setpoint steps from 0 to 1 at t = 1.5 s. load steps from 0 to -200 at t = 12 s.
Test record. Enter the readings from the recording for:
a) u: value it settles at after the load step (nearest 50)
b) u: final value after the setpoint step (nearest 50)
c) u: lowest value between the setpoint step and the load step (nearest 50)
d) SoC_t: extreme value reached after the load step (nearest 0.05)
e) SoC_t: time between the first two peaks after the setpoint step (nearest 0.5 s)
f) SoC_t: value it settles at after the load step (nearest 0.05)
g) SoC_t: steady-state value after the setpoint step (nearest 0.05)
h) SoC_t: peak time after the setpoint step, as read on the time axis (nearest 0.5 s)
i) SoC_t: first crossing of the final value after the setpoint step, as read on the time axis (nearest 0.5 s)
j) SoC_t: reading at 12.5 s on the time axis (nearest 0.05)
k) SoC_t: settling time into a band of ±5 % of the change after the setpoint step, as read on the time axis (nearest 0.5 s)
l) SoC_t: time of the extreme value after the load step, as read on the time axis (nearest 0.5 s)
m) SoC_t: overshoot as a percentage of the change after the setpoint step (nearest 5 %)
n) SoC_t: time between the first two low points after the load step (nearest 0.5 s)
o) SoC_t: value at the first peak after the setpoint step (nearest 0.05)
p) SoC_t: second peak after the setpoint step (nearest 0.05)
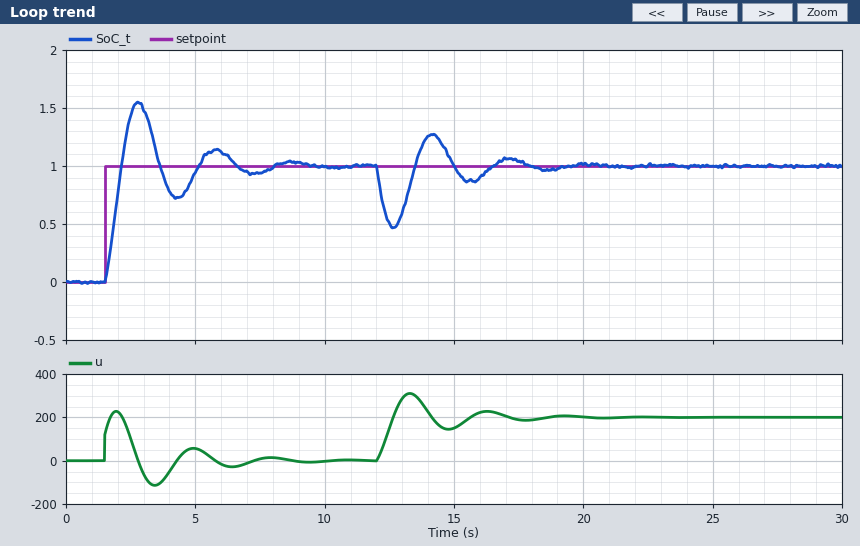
200
0
-100
0.45
3.0 s
1.00
1.00
3.0 s
2.0 s
0.50
7.5 s
12.5 s
55 %
3.0 s
1.55
1.15
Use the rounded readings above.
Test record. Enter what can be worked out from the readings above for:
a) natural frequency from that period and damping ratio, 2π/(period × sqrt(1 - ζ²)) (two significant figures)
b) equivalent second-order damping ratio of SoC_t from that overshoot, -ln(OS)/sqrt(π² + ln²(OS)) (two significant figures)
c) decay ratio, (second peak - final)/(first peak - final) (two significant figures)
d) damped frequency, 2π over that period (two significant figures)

2.1 rad/s
0.19
0.27
2.1 rad/s
